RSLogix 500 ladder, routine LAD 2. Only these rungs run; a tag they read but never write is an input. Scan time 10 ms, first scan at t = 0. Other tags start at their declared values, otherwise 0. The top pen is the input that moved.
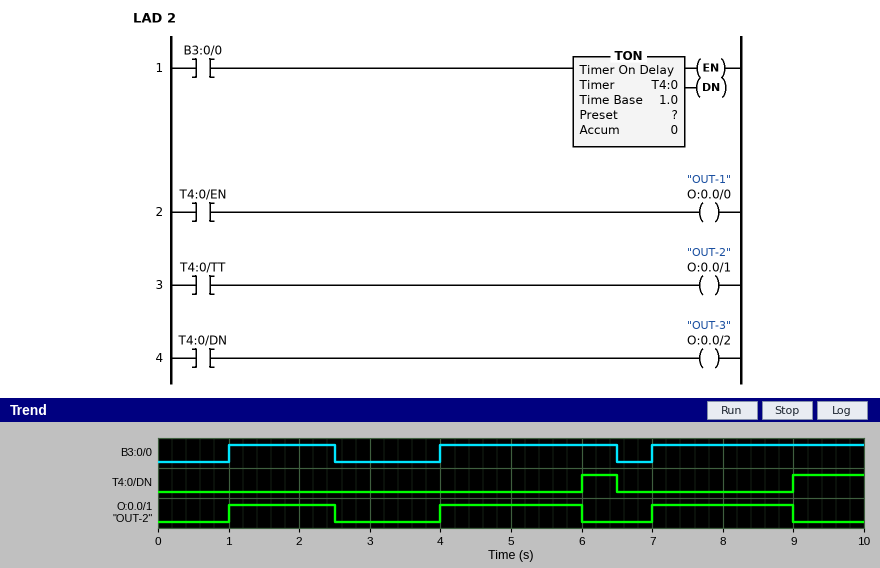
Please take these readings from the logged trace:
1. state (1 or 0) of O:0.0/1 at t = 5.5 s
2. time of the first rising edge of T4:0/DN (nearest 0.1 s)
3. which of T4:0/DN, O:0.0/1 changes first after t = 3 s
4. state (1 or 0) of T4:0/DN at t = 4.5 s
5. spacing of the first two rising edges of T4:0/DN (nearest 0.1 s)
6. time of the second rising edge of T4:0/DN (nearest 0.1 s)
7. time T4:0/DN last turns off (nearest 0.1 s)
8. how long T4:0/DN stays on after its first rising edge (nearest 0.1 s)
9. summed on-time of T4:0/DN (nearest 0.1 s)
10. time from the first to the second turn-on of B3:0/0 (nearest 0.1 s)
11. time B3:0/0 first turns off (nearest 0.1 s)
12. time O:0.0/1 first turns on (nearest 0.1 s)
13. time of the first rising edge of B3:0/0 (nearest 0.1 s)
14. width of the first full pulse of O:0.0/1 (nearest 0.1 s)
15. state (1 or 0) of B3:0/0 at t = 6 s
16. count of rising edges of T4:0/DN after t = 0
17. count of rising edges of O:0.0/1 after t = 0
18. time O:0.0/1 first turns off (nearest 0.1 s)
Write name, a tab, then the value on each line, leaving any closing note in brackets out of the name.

state (1 or 0) of O:0.0/1 at t = 5.5 s	1
time of the first rising edge of T4:0/DN	6.0 s
which of T4:0/DN, O:0.0/1 changes first after t = 3 s	O:0.0/1
state (1 or 0) of T4:0/DN at t = 4.5 s	0
spacing of the first two rising edges of T4:0/DN	3.0 s
time of the second rising edge of T4:0/DN	9.0 s
time T4:0/DN last turns off	6.5 s
how long T4:0/DN stays on after its first rising edge	0.5 s
summed on-time of T4:0/DN	1.5 s
time from the first to the second turn-on of B3:0/0	3.0 s
time B3:0/0 first turns off	2.5 s
time O:0.0/1 first turns on	1.0 s
time of the first rising edge of B3:0/0	1.0 s
width of the first full pulse of O:0.0/1	1.5 s
state (1 or 0) of B3:0/0 at t = 6 s	1
count of rising edges of T4:0/DN after t = 0	2
count of rising edges of O:0.0/1 after t = 0	3
time O:0.0/1 first turns off	2.5 s
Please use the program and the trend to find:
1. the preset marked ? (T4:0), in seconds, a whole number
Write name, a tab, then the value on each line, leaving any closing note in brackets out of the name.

the preset marked ? (T4:0), in seconds, a whole number	2 s
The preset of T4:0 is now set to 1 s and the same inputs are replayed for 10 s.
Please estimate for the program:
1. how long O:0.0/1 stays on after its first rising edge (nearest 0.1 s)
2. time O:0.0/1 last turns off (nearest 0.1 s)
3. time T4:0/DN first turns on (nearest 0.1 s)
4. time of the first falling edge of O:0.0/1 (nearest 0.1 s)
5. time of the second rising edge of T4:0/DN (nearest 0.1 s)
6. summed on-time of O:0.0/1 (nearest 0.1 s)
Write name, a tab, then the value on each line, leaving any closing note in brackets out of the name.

how long O:0.0/1 stays on after its first rising edge	1.0 s
time O:0.0/1 last turns off	8.0 s
time T4:0/DN first turns on	2.0 s
time of the first falling edge of O:0.0/1	2.0 s
time of the second rising edge of T4:0/DN	5.0 s
summed on-time of O:0.0/1	3.0 s
